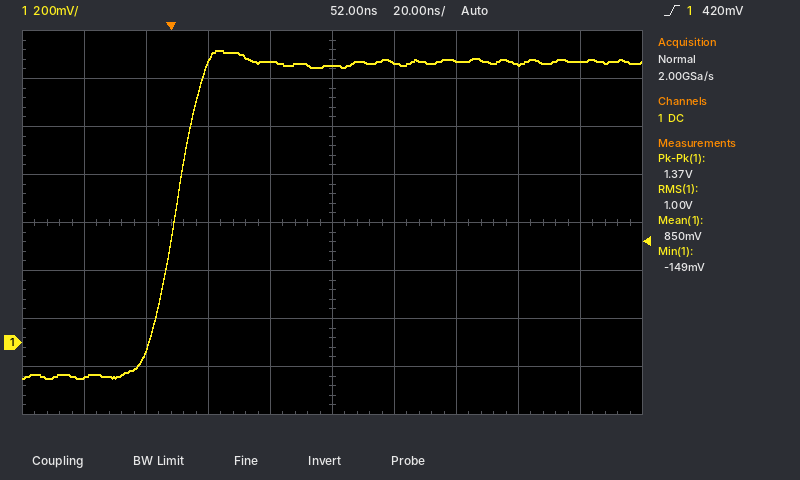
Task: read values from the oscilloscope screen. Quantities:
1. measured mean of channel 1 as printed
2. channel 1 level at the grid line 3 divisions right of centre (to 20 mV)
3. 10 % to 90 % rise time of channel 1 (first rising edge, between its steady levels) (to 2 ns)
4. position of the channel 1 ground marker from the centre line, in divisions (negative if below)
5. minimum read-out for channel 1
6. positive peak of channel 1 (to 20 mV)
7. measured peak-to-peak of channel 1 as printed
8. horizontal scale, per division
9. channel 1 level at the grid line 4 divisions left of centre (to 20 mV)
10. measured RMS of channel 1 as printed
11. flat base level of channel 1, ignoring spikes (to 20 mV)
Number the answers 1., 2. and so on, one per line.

1. 850 mV
2. 1.16 V
3. 16 ns
4. -2.5 div
5. -149 mV
6. 1.22 V
7. 1.37 V
8. 20 ns
9. -140 mV
10. 1.00 V
11. -140 mV
